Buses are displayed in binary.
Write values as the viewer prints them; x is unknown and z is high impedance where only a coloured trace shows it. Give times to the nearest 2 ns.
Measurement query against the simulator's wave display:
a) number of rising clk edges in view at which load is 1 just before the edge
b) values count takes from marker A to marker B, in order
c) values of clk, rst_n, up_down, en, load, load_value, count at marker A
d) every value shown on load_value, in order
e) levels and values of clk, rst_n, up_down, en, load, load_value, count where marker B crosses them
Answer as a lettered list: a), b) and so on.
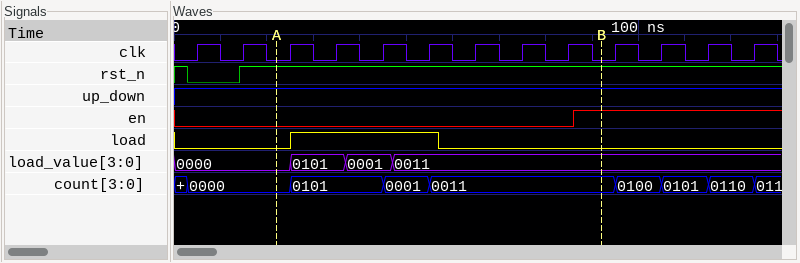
a) 3
b) 0000, 0101, 0001, 0011
c) clk=0, rst_n=1, up_down=1, en=0, load=0, load_value=0000, count=0000
d) 0000, 0101, 0001, 0011
e) clk=0, rst_n=1, up_down=1, en=1, load=0, load_value=0011, count=0011
